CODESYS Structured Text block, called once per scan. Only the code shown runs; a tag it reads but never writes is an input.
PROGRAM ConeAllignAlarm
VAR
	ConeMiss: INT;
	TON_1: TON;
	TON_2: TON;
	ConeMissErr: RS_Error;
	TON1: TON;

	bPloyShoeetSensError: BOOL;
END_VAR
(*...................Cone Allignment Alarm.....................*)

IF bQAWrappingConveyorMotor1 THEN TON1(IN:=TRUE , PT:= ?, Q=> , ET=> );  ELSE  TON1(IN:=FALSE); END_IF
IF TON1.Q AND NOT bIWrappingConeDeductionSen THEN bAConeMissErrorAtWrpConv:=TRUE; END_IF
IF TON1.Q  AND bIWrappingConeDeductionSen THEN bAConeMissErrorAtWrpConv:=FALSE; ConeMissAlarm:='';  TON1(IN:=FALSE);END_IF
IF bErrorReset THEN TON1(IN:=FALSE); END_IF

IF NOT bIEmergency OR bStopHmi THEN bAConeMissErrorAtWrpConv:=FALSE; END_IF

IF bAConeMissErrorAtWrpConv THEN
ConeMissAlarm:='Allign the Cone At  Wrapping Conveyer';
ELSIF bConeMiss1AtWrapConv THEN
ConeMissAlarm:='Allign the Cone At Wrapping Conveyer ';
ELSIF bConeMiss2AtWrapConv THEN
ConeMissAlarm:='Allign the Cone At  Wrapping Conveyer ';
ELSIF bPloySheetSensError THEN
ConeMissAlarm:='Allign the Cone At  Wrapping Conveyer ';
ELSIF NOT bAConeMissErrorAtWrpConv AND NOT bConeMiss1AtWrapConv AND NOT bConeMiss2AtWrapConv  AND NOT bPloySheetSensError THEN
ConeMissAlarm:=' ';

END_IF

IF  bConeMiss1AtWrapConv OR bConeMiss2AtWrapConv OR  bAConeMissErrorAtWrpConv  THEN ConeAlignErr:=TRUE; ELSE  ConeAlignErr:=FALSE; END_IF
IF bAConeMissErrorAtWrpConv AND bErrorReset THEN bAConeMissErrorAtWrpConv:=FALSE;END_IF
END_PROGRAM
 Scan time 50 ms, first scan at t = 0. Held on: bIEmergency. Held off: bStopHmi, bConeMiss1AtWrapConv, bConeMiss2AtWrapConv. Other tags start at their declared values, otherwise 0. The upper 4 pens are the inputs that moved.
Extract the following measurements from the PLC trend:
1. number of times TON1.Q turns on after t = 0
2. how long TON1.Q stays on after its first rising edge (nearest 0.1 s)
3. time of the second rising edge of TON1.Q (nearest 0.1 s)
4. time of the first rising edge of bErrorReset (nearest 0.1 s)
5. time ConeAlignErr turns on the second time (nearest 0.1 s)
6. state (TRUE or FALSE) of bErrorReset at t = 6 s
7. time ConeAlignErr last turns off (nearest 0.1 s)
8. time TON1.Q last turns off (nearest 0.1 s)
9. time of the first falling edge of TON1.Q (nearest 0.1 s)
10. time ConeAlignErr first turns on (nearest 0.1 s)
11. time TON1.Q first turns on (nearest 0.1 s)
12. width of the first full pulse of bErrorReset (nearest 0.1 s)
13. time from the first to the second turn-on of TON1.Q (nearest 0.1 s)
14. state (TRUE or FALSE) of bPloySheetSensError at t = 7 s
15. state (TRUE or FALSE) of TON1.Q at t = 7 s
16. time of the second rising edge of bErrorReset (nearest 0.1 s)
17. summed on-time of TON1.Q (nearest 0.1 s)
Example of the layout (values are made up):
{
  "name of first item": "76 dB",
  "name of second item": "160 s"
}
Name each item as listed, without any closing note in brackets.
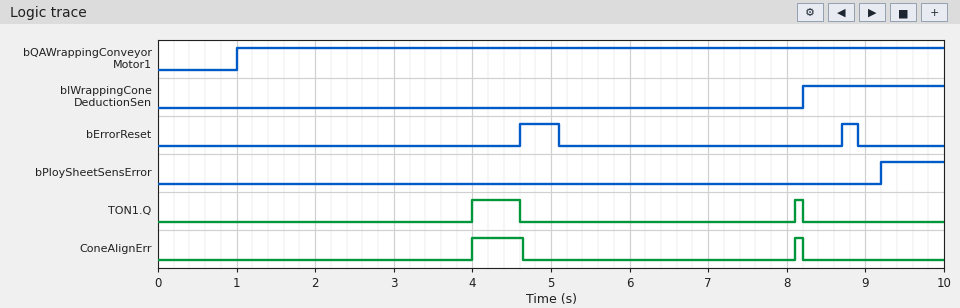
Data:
{
  "number of times TON1.Q turns on after t = 0": "2",
  "how long TON1.Q stays on after its first rising edge": "0.6 s",
  "time of the second rising edge of TON1.Q": "8.1 s",
  "time of the first rising edge of bErrorReset": "4.6 s",
  "time ConeAlignErr turns on the second time": "8.1 s",
  "state (TRUE or FALSE) of bErrorReset at t = 6 s": "FALSE",
  "time ConeAlignErr last turns off": "8.2 s",
  "time TON1.Q last turns off": "8.2 s",
  "time of the first falling edge of TON1.Q": "4.6 s",
  "time ConeAlignErr first turns on": "4.0 s",
  "time TON1.Q first turns on": "4.0 s",
  "width of the first full pulse of bErrorReset": "0.5 s",
  "time from the first to the second turn-on of TON1.Q": "4.1 s",
  "state (TRUE or FALSE) of bPloySheetSensError at t = 7 s": "FALSE",
  "state (TRUE or FALSE) of TON1.Q at t = 7 s": "FALSE",
  "time of the second rising edge of bErrorReset": "8.7 s",
  "summed on-time of TON1.Q": "0.7 s"
}
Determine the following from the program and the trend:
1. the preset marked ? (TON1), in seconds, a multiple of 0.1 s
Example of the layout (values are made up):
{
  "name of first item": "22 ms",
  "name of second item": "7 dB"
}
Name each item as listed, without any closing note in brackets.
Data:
{
  "the preset marked ? (TON1), in seconds, a multiple of 0.1 s": "3.0 s"
}
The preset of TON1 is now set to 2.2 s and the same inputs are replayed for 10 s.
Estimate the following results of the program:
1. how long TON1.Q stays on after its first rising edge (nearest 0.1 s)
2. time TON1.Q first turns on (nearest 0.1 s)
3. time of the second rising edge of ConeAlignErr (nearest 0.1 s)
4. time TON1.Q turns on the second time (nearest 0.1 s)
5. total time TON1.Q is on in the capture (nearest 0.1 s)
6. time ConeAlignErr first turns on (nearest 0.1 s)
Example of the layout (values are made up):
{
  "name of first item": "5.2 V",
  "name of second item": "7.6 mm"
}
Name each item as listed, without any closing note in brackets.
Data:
{
  "how long TON1.Q stays on after its first rising edge": "1.4 s",
  "time TON1.Q first turns on": "3.2 s",
  "time of the second rising edge of ConeAlignErr": "7.3 s",
  "time TON1.Q turns on the second time": "7.3 s",
  "total time TON1.Q is on in the capture": "2.3 s",
  "time ConeAlignErr first turns on": "3.2 s"
}
